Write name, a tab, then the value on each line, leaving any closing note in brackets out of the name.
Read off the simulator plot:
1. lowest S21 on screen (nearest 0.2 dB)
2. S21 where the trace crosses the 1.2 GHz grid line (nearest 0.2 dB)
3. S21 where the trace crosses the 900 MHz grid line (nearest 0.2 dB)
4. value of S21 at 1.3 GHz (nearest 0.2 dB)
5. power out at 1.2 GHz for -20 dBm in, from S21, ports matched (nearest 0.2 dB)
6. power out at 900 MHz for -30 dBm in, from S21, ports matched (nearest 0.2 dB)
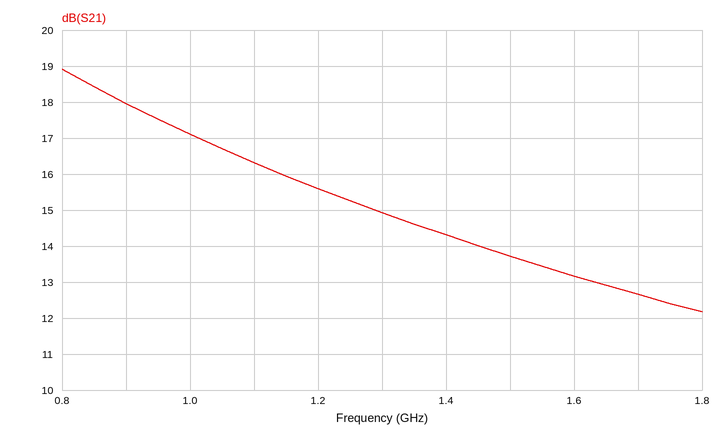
lowest S21 on screen	12.2 dB
S21 where the trace crosses the 1.2 GHz grid line	15.6 dB
S21 where the trace crosses the 900 MHz grid line	18.0 dB
value of S21 at 1.3 GHz	15.0 dB
power out at 1.2 GHz for -20 dBm in, from S21, ports matched	-4.4 dBm
power out at 900 MHz for -30 dBm in, from S21, ports matched	-12.0 dBm
